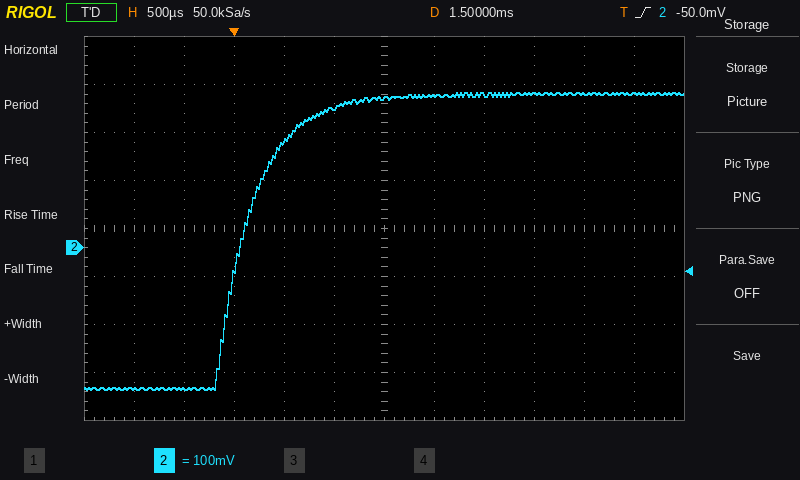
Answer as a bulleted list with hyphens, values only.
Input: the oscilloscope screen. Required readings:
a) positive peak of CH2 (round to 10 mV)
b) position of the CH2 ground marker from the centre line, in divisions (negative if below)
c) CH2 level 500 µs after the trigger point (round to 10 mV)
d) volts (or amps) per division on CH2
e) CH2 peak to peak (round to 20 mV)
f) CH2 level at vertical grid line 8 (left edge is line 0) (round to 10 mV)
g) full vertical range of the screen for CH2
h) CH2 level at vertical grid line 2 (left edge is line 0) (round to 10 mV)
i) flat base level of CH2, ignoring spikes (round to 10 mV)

- 320 mV
- -0.4 div
- 220 mV
- 100 mV
- 620 mV
- 320 mV
- 800 mV
- -290 mV
- -290 mV
